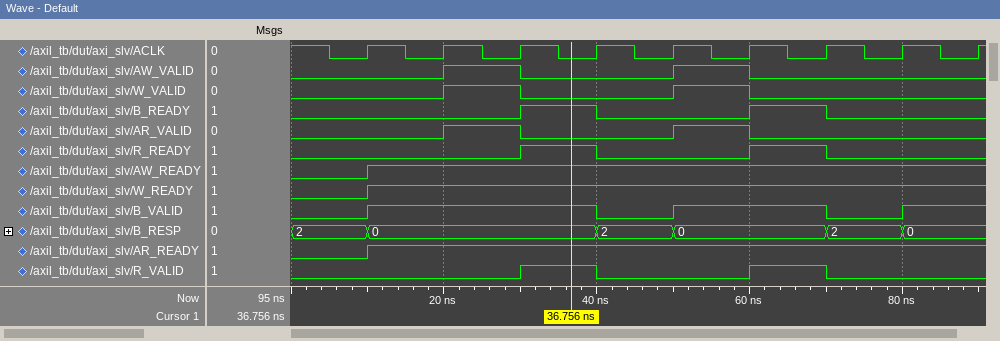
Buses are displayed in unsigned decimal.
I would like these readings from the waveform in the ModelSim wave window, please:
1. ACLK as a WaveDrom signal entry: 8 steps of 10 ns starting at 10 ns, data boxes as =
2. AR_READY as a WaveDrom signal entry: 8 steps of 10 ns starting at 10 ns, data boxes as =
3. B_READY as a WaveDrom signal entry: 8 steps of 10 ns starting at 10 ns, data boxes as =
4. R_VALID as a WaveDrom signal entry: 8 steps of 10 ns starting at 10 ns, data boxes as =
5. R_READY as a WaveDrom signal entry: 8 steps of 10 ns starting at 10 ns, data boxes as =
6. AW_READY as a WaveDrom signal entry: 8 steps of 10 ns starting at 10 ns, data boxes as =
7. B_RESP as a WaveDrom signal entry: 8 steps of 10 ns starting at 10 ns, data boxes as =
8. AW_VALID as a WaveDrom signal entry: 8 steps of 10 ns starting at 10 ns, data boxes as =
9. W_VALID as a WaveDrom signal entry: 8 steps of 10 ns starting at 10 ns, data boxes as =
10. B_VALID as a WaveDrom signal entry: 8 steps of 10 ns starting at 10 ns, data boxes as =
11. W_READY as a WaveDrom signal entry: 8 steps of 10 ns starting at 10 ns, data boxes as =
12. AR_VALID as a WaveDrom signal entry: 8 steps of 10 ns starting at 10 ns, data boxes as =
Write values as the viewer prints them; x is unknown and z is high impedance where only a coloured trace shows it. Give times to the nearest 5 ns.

{name: 'ACLK', wave: 'p.......'}
{name: 'AR_READY', wave: '1.......'}
{name: 'B_READY', wave: '0.10.10.'}
{name: 'R_VALID', wave: '0.10.10.'}
{name: 'R_READY', wave: '0.10.10.'}
{name: 'AW_READY', wave: '1.......'}
{name: 'B_RESP', wave: '=..==.==', data: '0 2 0 2 0'}
{name: 'AW_VALID', wave: '010.10..'}
{name: 'W_VALID', wave: '010.10..'}
{name: 'B_VALID', wave: '1..01.01'}
{name: 'W_READY', wave: '1.......'}
{name: 'AR_VALID', wave: '010.10..'}
